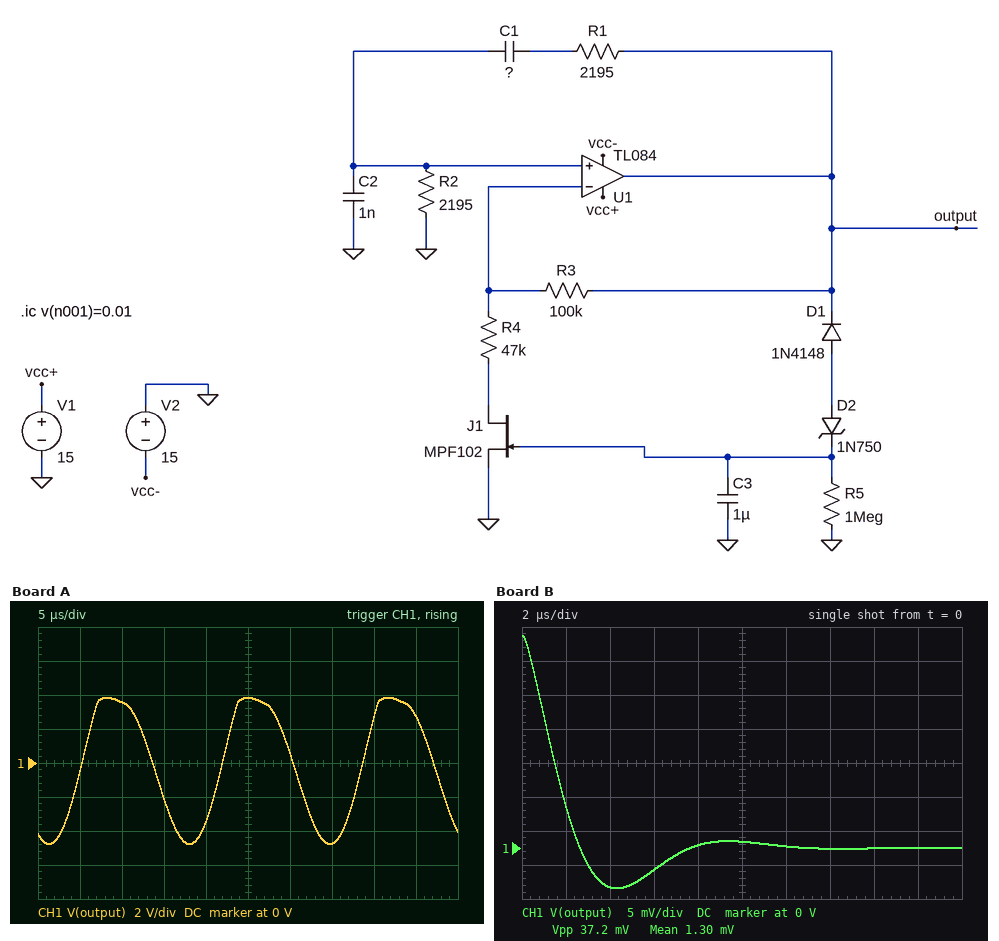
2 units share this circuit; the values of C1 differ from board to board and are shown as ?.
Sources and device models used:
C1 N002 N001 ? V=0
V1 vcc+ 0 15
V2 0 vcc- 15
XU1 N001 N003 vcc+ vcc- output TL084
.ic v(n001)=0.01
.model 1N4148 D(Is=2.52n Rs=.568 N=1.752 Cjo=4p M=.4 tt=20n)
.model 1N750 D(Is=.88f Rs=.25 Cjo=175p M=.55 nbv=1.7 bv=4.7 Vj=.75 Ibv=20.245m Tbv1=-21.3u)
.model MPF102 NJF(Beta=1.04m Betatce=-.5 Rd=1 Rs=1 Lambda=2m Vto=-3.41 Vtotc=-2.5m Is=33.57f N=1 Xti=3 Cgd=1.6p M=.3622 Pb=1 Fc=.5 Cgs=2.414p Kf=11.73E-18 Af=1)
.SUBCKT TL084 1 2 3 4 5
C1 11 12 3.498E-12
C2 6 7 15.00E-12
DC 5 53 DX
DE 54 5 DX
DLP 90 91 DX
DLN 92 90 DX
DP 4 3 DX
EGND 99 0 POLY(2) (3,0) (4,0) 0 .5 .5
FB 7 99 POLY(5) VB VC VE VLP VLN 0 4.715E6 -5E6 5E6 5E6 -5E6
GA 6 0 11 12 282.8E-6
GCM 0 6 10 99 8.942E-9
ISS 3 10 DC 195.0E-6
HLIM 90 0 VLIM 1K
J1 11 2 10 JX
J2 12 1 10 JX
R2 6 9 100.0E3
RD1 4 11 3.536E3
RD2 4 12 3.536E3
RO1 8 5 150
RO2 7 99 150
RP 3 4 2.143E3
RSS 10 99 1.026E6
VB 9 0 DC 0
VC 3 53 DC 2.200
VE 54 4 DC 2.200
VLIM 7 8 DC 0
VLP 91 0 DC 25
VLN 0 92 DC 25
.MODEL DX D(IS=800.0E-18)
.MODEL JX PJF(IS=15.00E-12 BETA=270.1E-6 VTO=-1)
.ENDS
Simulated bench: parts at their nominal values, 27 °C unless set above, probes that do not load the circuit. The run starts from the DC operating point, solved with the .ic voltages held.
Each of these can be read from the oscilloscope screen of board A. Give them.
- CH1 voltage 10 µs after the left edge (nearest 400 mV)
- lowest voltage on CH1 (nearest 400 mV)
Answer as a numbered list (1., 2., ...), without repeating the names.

1. 3.6 V
2. -4.8 V
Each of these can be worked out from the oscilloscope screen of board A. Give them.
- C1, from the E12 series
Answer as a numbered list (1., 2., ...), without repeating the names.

1. 1.2 nF
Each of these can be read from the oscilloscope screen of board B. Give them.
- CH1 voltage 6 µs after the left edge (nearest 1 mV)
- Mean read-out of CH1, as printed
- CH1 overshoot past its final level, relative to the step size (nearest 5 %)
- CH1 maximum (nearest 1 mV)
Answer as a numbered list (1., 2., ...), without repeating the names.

1. -3 mV
2. 1.30 mV
3. 20 %
4. 31 mV
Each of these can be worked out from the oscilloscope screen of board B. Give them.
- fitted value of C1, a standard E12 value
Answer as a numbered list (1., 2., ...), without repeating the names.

1. 330 pF
